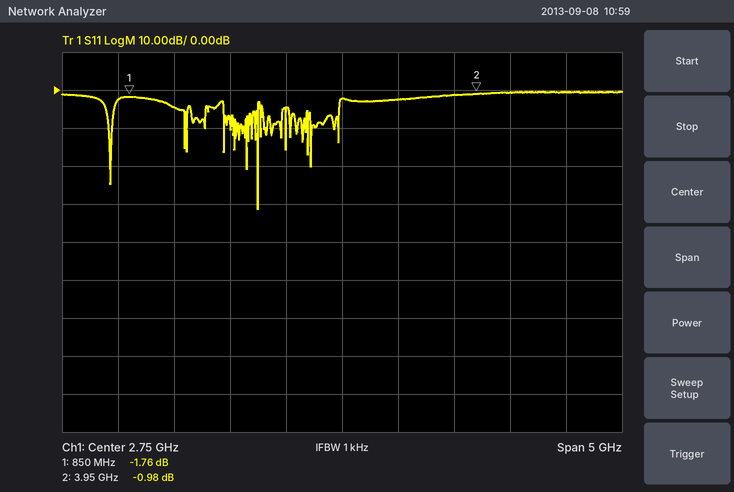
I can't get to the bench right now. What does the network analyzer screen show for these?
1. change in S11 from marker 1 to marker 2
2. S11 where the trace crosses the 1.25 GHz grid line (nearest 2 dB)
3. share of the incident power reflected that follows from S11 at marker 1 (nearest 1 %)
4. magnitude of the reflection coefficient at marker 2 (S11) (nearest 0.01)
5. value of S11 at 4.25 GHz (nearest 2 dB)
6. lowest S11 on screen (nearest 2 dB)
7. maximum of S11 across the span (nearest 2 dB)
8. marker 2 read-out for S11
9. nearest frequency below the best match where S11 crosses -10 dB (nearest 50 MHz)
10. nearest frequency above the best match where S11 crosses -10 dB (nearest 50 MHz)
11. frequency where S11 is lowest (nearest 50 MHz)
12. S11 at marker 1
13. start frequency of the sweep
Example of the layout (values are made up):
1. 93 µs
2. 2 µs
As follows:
1. 0.78 dB
2. -4 dB
3. 67 %
4. 0.89
5. 0 dB
6. -32 dB
7. 0 dB
8. -0.98 dB
9. 2.00 GHz
10. 2.00 GHz
11. 2.00 GHz
12. -1.76 dB
13. 250 MHz
